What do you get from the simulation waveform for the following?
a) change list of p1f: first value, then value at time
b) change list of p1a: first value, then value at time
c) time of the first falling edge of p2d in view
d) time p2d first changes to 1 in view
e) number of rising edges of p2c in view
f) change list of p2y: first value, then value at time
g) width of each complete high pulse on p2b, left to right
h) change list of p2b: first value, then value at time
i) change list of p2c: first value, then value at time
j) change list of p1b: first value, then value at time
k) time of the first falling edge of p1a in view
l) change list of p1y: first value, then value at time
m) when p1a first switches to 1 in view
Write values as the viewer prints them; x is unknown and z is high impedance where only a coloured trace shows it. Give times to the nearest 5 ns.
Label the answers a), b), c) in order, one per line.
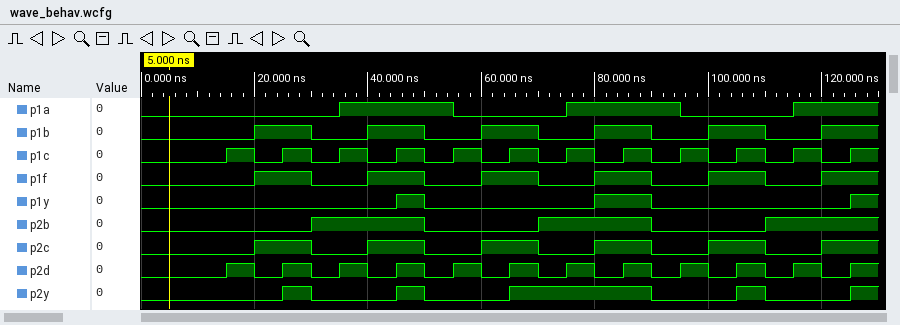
a) 0, 1 at 20 ns, 0 at 30 ns, 1 at 40 ns, 0 at 50 ns, 1 at 60 ns, 0 at 70 ns, 1 at 80 ns, 0 at 90 ns, 1 at 100 ns, 0 at 110 ns, 1 at 120 ns
b) 0, 1 at 35 ns, 0 at 55 ns, 1 at 75 ns, 0 at 95 ns, 1 at 115 ns
c) 20 ns
d) 15 ns
e) 6
f) 0, 1 at 25 ns, 0 at 30 ns, 1 at 45 ns, 0 at 50 ns, 1 at 65 ns, 0 at 90 ns, 1 at 105 ns, 0 at 110 ns, 1 at 125 ns
g) 20 ns, 20 ns
h) 0, 1 at 30 ns, 0 at 50 ns, 1 at 70 ns, 0 at 90 ns, 1 at 110 ns
i) 0, 1 at 20 ns, 0 at 30 ns, 1 at 40 ns, 0 at 50 ns, 1 at 60 ns, 0 at 70 ns, 1 at 80 ns, 0 at 90 ns, 1 at 100 ns, 0 at 110 ns, 1 at 120 ns
j) 0, 1 at 20 ns, 0 at 30 ns, 1 at 40 ns, 0 at 50 ns, 1 at 60 ns, 0 at 70 ns, 1 at 80 ns, 0 at 90 ns, 1 at 100 ns, 0 at 110 ns, 1 at 120 ns
k) 55 ns
l) 0, 1 at 45 ns, 0 at 50 ns, 1 at 80 ns, 0 at 90 ns, 1 at 125 ns
m) 35 ns
